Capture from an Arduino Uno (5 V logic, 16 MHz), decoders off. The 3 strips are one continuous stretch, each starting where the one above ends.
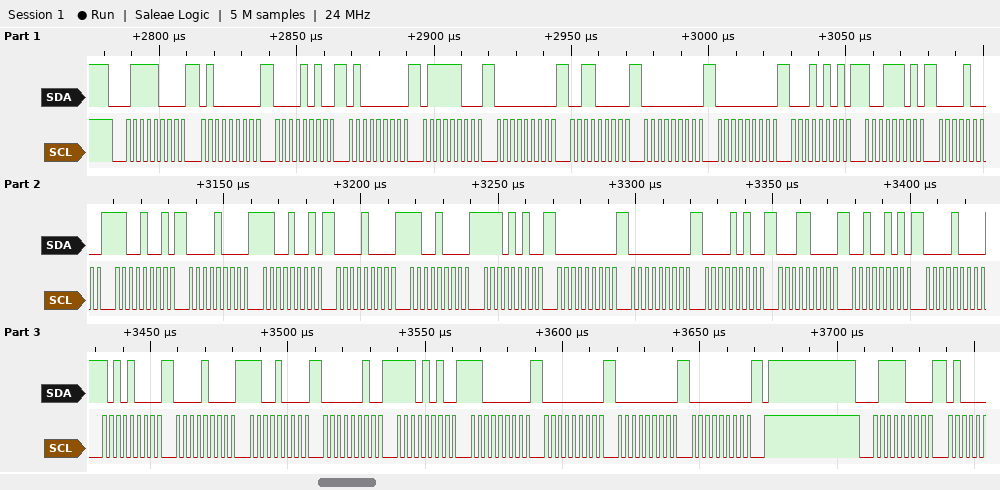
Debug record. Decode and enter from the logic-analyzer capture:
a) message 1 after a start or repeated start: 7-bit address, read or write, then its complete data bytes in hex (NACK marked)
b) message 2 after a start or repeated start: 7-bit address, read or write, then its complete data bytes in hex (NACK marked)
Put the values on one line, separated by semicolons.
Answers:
0x3C write: 40 0A 40 7C 00 30 00 00 15 9D 08 C9 08 C9 08 C8 EA 00 00 0A 18 25 08 A8 08 C8 02 EA C0 00 00 00; 0x3C write
